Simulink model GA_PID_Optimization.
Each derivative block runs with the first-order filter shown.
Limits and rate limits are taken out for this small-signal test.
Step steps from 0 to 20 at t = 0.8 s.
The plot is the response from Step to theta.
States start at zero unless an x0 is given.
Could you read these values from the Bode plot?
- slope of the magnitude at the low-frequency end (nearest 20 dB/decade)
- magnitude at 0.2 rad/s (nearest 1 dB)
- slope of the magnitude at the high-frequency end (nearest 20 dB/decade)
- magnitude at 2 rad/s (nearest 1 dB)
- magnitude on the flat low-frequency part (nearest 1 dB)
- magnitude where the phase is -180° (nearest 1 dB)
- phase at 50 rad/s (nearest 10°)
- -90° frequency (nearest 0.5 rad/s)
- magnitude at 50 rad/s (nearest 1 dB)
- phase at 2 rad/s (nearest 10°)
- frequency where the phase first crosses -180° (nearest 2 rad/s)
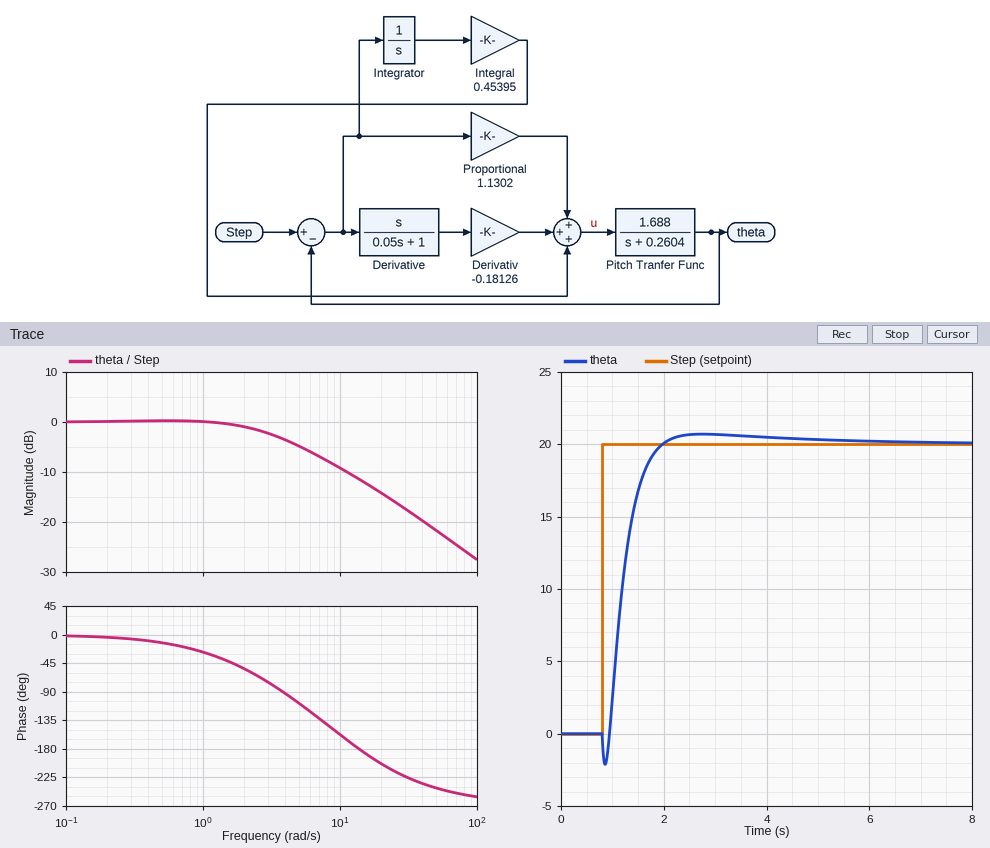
0 dB/decade
0 dB
-20 dB/decade
-1 dB
0 dB
-11 dB
-240°
4.0 rad/s
-22 dB
-50°
14 rad/s
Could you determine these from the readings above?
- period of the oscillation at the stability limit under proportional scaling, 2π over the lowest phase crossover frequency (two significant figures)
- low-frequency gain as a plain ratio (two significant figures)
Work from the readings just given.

0.45 s
1.0
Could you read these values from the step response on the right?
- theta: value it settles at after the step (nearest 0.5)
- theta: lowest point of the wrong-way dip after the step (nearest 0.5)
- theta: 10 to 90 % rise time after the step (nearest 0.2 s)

20.0
-2.0
0.6 s
